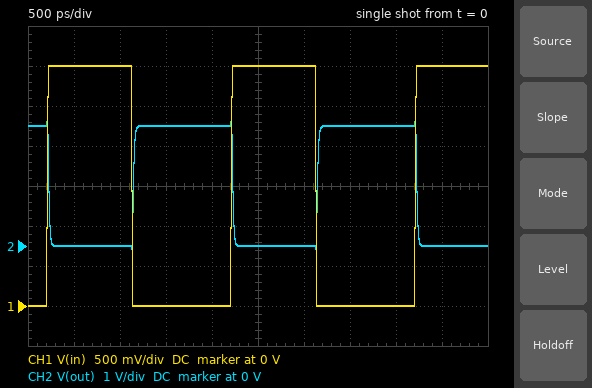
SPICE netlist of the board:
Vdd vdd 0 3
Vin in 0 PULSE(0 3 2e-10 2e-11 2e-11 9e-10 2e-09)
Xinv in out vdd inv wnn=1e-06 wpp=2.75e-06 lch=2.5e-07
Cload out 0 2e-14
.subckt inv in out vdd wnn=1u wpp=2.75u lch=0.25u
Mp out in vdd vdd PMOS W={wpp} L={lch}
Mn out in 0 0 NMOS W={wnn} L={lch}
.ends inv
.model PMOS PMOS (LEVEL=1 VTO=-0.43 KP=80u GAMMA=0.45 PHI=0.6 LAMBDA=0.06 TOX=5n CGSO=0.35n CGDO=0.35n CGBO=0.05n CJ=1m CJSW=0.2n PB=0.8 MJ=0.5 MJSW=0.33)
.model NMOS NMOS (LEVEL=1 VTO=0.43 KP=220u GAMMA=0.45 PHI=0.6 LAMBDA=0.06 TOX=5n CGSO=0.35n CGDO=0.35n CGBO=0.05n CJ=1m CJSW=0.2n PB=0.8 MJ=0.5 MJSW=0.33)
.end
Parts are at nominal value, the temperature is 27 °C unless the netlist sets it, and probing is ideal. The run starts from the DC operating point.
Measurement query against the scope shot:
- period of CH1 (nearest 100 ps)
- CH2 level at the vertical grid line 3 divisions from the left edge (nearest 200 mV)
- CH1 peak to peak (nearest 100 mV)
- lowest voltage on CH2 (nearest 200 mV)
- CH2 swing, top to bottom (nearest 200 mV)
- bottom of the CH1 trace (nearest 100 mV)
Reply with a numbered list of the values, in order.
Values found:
1. 2.0 ns
2. 3.0 V
3. 3.0 V
4. 0 V
5. 3.2 V
6. 0 V
